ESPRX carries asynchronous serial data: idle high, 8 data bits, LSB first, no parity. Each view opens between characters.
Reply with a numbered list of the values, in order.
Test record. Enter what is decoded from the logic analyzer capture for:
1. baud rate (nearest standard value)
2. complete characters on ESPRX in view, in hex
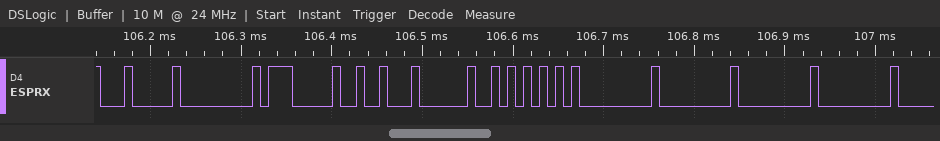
1. 115200 baud
2. 04, 00, 07, 12, 20, 55, 00, 00, 00, 00
